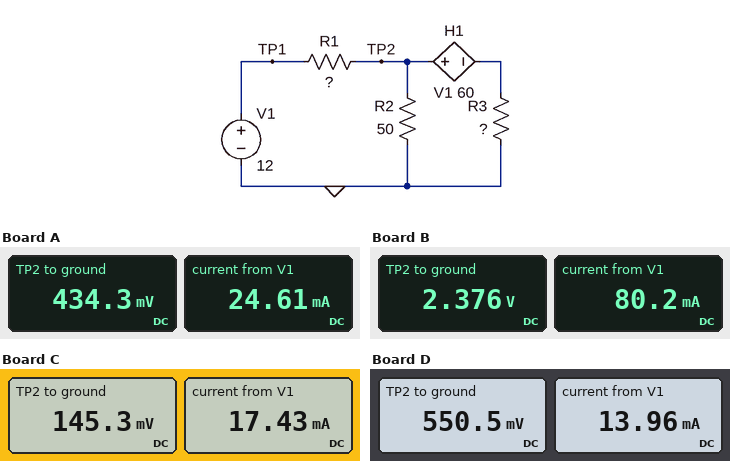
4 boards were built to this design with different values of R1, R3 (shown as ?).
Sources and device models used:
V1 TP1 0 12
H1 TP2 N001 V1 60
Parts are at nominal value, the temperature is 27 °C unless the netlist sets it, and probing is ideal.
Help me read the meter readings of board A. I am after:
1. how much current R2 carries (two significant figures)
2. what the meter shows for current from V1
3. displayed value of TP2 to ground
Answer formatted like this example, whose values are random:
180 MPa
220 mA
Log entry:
8.7 mA
24.61 mA
434.3 mV
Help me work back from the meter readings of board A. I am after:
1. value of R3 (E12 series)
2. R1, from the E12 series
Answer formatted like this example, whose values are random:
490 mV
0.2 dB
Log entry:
120 Ω
470 Ω
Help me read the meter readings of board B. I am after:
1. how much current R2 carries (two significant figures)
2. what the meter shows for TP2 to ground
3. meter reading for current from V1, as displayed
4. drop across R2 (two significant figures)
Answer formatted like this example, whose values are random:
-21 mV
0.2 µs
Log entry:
48 mA
2.376 V
80.2 mA
2.4 V
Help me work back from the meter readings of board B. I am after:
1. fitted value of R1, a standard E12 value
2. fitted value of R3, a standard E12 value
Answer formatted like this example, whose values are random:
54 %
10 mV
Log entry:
120 Ω
220 Ω
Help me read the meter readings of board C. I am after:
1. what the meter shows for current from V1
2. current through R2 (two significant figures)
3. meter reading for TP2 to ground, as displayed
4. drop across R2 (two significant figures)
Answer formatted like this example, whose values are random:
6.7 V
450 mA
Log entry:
17.43 mA
2.9 mA
145.3 mV
150 mV
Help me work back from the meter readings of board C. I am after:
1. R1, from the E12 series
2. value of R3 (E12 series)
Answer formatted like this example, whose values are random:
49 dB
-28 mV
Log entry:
680 Ω
82 Ω
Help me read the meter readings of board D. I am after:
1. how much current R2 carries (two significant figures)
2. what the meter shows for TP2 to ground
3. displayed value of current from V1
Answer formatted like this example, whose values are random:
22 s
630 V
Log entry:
11 mA
550.5 mV
13.96 mA
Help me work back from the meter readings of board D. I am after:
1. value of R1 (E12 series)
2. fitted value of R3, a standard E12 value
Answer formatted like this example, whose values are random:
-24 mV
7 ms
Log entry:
820 Ω
470 Ω
